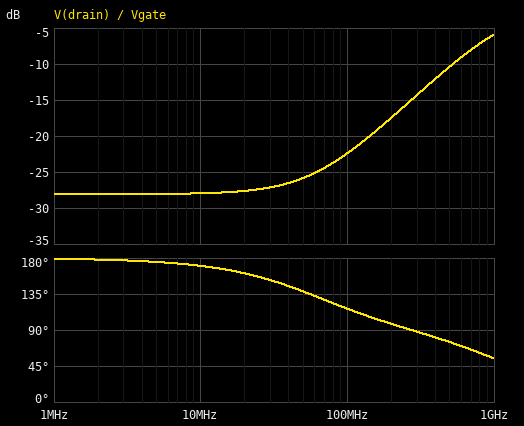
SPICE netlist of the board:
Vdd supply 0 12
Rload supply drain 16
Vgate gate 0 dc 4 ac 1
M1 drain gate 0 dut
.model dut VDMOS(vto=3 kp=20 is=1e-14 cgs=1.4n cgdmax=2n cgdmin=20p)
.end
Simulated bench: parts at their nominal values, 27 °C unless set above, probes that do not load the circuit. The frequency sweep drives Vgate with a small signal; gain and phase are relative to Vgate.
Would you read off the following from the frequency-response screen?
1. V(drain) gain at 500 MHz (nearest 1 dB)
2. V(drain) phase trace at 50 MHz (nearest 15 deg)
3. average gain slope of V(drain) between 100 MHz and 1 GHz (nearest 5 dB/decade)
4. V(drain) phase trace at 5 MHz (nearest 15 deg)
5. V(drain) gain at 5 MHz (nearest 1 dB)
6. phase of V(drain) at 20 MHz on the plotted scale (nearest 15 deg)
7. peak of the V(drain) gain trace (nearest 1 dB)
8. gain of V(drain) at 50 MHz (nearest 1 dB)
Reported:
-10 dB
135 deg
15 dB/decade
180 deg
-28 dB
165 deg
-6 dB
-26 dB
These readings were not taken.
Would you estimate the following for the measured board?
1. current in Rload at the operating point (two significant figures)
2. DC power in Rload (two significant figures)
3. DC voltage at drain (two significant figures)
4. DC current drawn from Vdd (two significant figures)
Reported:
750 mA
8.9 W
38 mV
750 mA
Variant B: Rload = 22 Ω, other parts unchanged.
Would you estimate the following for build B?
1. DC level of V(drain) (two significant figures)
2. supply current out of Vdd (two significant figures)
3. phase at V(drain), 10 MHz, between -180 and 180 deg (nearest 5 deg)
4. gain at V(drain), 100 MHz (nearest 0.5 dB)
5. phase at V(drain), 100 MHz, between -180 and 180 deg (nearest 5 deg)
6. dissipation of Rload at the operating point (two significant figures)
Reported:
28 mV
540 mA
165 deg
-23.0 dB
110 deg
6.5 W
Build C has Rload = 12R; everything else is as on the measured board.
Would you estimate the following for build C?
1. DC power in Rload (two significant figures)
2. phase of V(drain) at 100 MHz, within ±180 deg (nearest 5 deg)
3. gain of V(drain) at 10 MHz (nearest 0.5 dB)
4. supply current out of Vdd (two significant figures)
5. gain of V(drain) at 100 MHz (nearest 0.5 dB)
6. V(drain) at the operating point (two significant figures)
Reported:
12 W
125 deg
-25.5 dB
1.0 A
-21.5 dB
51 mV
